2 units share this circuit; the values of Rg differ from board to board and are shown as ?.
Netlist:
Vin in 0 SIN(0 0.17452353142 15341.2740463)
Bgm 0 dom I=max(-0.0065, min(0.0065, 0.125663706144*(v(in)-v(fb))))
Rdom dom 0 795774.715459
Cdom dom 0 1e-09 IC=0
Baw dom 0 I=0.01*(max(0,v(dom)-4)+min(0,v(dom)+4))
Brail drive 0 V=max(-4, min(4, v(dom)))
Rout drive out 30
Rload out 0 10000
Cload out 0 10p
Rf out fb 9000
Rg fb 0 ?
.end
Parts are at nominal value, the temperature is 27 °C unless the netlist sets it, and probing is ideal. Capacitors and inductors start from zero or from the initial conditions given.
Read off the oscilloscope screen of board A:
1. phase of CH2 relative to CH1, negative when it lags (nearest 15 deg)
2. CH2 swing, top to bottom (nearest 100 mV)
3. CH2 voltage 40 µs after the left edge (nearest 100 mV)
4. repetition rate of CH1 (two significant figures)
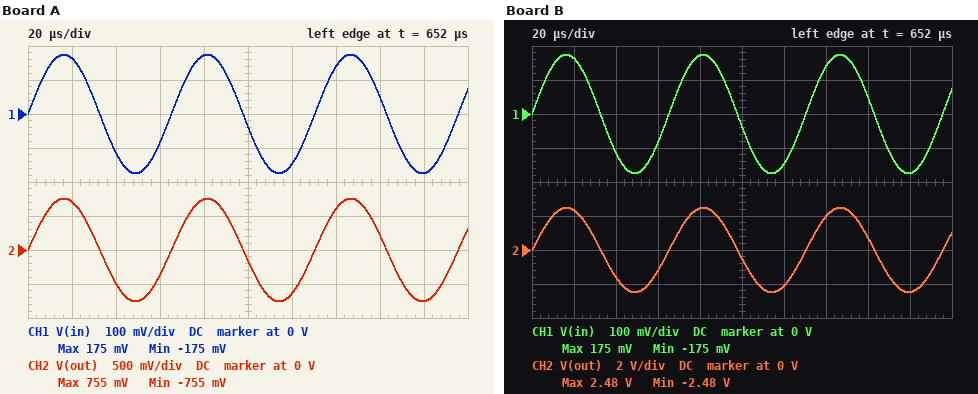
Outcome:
0 deg
1.5 V
-500 mV
15 kHz
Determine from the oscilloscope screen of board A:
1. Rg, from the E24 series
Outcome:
2.7 kΩ
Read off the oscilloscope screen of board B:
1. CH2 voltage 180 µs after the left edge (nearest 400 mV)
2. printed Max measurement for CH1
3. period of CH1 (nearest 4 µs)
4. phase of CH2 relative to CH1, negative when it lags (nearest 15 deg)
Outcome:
-2.4 V
175 mV
64 µs
0 deg
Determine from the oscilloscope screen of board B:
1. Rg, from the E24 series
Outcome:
680 Ω
